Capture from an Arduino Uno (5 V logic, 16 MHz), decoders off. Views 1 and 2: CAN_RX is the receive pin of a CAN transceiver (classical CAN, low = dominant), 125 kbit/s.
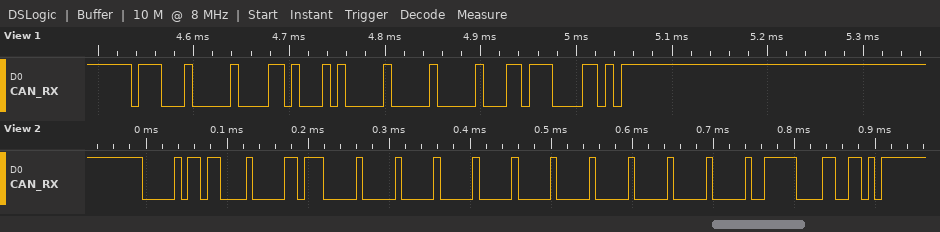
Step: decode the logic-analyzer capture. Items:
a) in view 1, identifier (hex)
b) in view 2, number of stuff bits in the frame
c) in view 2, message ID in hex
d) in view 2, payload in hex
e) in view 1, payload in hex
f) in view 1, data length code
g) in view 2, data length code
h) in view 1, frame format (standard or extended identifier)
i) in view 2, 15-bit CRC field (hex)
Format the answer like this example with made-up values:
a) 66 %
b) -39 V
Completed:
a) 0x710
b) 14
c) 0x036
d) 2E 00 00 00 00 00 00 00
e) 45 00 00
f) 3
g) 8
h) standard
i) 0x7C66
